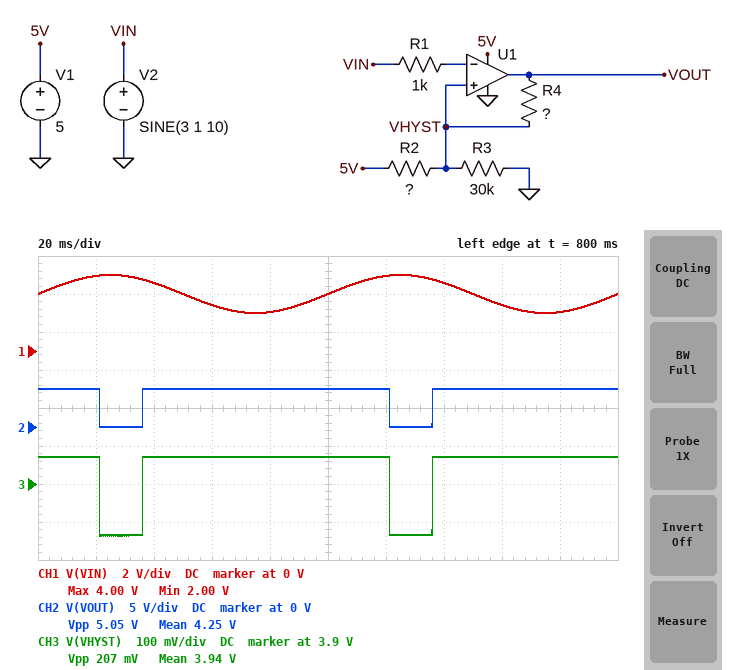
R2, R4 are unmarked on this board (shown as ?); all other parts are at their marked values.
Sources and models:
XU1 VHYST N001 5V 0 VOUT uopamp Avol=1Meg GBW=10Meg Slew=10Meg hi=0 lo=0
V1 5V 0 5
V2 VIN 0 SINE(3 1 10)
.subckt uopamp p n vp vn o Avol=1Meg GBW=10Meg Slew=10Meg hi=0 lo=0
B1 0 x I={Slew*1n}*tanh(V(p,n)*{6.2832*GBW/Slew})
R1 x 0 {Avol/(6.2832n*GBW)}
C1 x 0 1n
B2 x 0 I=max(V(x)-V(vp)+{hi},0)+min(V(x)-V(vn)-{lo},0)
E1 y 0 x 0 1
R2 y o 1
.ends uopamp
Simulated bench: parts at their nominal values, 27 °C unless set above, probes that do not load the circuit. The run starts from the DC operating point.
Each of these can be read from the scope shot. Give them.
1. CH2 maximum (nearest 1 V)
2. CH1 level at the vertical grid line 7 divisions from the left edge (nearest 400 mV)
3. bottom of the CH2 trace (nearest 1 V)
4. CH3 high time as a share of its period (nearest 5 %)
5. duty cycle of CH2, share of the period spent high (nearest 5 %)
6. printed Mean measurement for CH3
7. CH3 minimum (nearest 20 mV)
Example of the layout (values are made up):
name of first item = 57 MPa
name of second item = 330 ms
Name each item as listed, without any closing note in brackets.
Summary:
CH2 maximum = 5 V
CH1 level at the vertical grid line 7 divisions from the left edge = 3.6 V
bottom of the CH2 trace = 0 V
CH3 high time as a share of its period = 85 %
duty cycle of CH2, share of the period spent high = 85 %
printed Mean measurement for CH3 = 3.94 V
CH3 minimum = 3.76 V
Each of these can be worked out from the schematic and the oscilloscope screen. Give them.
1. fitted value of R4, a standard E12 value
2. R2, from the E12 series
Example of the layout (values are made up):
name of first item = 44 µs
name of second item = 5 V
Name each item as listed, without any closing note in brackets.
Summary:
fitted value of R4, a standard E12 value = 150 kΩ
R2, from the E12 series = 8.2 kΩ
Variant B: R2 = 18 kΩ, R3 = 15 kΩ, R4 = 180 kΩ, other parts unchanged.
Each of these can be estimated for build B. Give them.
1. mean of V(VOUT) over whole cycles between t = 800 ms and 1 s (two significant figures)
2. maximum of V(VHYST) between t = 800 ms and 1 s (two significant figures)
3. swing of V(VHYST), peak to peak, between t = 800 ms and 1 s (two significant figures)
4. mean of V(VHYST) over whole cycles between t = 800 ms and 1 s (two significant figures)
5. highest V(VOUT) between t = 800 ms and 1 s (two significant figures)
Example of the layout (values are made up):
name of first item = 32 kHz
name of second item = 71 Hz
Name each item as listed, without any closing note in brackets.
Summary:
mean of V(VOUT) over whole cycles between t = 800 ms and 1 s = 1.2 V
maximum of V(VHYST) between t = 800 ms and 1 s = 2.4 V
swing of V(VHYST), peak to peak, between t = 800 ms and 1 s = 220 mV
mean of V(VHYST) over whole cycles between t = 800 ms and 1 s = 2.2 V
highest V(VOUT) between t = 800 ms and 1 s = 5.0 V
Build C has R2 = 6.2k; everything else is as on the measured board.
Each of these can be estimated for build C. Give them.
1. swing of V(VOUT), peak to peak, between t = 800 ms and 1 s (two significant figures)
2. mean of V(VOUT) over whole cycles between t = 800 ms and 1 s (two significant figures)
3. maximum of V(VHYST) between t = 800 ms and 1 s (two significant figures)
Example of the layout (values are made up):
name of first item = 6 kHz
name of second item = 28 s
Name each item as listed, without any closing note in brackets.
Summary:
swing of V(VOUT), peak to peak, between t = 800 ms and 1 s = 2.1 mV
mean of V(VOUT) over whole cycles between t = 800 ms and 1 s = 5.0 V
maximum of V(VHYST) between t = 800 ms and 1 s = 4.2 V
